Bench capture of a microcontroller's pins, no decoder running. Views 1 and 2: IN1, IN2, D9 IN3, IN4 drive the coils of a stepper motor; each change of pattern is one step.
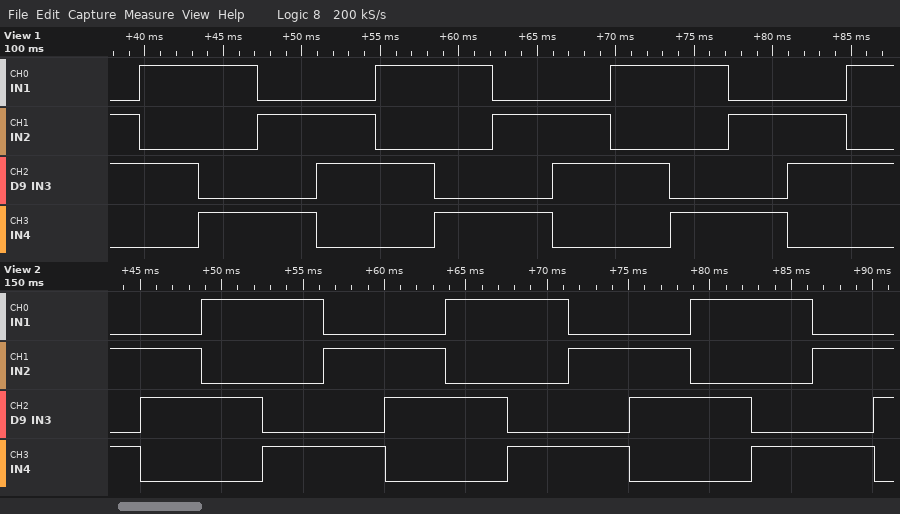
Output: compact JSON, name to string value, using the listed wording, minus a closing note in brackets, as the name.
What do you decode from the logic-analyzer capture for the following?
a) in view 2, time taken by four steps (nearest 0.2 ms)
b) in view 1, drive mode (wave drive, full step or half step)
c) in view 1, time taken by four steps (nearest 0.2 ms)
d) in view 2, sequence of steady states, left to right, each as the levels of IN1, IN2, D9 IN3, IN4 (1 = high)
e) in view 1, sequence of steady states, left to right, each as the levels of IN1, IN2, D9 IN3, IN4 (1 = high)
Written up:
{"in view 2, time taken by four steps": "15.0 ms", "in view 1, drive mode": "full step", "in view 1, time taken by four steps": "15.0 ms", "in view 2, sequence of steady states, left to right, each as the levels of IN1, IN2, D9 IN3, IN4": "0101 0110 1010 1001 0101 0110 1010 1001 0101 0110 1010 1001 0101 0110", "in view 1, sequence of steady states, left to right, each as the levels of IN1, IN2, D9 IN3, IN4": "0110 1010 1001 0101 0110 1010 1001 0101 0110 1010 1001 0101 0110 1010"}
